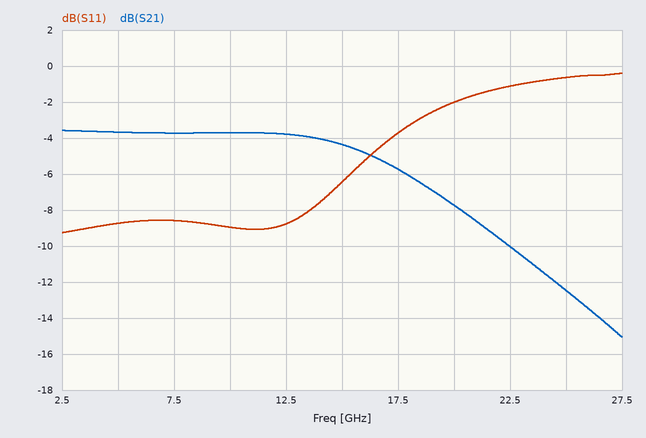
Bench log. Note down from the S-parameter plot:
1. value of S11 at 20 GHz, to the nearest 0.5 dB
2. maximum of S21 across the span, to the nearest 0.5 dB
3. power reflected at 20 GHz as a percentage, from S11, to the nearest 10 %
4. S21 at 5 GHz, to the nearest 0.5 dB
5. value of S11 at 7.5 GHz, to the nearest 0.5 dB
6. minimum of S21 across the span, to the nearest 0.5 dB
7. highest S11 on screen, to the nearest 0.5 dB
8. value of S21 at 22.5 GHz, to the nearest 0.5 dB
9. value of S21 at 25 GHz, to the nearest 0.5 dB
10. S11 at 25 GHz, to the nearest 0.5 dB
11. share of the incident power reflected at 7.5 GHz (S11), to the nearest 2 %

-2.0 dB
-3.5 dB
60 %
-3.5 dB
-8.5 dB
-15.0 dB
-0.5 dB
-10.0 dB
-12.5 dB
-0.5 dB
14 %
